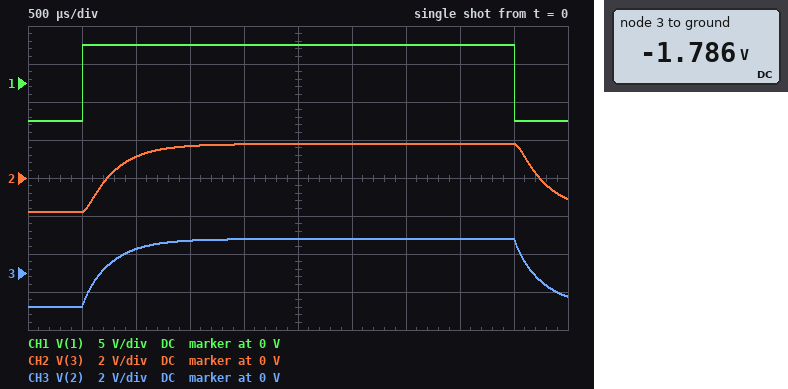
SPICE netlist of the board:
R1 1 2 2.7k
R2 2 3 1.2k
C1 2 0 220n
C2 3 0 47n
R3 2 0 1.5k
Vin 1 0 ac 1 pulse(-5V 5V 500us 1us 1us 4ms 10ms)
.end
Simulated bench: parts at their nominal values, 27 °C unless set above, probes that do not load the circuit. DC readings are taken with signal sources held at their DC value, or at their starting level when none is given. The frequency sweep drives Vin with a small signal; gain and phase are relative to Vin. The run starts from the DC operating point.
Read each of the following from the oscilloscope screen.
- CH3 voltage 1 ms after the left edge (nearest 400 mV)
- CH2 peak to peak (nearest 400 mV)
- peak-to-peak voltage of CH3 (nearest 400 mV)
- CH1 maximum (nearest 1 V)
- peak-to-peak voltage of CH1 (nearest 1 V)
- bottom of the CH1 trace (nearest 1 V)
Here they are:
1.2 V
3.6 V
3.6 V
5 V
10 V
-5 V
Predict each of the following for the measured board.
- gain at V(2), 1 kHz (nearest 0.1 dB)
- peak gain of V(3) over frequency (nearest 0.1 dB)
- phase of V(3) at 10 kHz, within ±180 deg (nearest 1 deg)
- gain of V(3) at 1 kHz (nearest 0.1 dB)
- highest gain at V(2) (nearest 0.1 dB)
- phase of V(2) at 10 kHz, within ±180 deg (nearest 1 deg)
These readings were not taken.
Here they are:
-14.6 dB
-8.9 dB
-157 deg
-15.1 dB
-8.9 dB
-83 deg
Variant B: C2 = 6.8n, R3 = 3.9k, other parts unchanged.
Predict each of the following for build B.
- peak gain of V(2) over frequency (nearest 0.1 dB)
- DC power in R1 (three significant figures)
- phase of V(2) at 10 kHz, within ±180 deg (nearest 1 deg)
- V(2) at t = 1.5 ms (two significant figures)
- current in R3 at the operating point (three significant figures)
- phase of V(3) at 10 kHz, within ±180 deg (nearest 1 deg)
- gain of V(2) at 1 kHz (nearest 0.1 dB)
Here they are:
-4.6 dB
1.55 mW
-87 deg
2.6 V
758 µA
-114 deg
-12.5 dB
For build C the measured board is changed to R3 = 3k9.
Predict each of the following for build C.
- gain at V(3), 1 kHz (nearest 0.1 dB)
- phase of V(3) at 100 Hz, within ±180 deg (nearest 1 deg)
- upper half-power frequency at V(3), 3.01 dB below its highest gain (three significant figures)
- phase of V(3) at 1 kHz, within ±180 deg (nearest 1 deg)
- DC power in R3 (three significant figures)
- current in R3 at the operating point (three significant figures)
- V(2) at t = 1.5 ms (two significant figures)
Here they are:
-14.2 dB
-17 deg
360 Hz
-86 deg
2.24 mW
758 µA
2.4 V
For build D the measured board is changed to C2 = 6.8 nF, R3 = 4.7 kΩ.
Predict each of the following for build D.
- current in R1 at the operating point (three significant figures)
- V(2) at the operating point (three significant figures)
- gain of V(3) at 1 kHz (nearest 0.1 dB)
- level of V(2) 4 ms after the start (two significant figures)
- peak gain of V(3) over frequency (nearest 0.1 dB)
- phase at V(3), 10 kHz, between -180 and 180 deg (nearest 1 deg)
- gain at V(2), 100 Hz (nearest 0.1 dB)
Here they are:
676 µA
-3.18 V
-12.4 dB
3.2 V
-3.9 dB
-114 deg
-4.2 dB
